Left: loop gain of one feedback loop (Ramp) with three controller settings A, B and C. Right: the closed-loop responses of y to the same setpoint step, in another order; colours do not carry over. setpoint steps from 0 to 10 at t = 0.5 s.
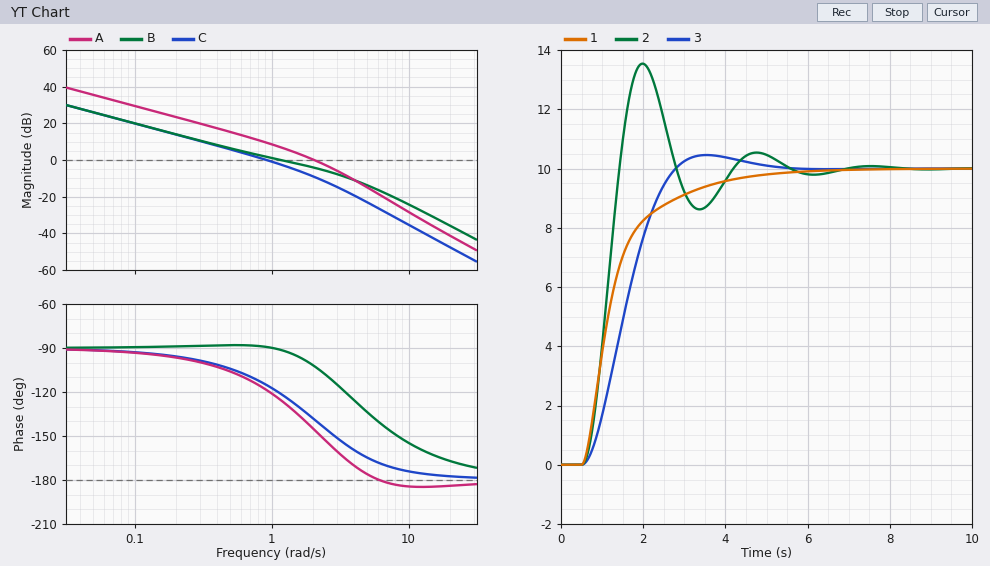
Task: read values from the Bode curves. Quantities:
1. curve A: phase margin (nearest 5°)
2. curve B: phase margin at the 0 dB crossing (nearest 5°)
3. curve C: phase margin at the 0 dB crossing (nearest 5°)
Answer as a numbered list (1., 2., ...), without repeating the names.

1. 35°
2. 90°
3. 65°
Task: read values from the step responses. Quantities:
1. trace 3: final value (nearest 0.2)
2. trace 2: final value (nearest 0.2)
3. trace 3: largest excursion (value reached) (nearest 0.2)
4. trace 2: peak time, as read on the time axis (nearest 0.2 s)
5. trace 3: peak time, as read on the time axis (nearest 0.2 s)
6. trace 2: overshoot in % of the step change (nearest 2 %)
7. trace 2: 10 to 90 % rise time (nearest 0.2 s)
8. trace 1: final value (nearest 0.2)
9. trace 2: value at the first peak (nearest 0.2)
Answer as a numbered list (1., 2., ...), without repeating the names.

1. 10.0
2. 10.0
3. 10.4
4. 2.0 s
5. 3.6 s
6. 36 %
7. 0.6 s
8. 10.0
9. 13.6
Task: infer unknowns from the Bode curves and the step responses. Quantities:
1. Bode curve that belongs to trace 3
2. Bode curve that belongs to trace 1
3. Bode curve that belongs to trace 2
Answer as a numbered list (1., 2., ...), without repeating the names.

1. C
2. B
3. A
